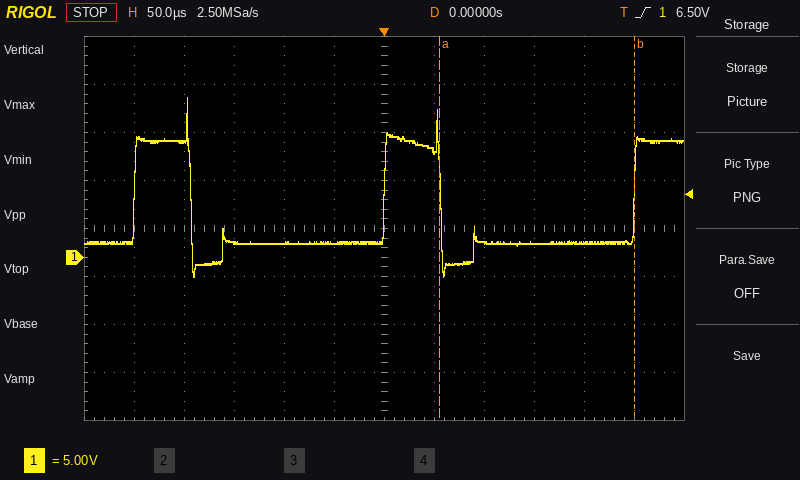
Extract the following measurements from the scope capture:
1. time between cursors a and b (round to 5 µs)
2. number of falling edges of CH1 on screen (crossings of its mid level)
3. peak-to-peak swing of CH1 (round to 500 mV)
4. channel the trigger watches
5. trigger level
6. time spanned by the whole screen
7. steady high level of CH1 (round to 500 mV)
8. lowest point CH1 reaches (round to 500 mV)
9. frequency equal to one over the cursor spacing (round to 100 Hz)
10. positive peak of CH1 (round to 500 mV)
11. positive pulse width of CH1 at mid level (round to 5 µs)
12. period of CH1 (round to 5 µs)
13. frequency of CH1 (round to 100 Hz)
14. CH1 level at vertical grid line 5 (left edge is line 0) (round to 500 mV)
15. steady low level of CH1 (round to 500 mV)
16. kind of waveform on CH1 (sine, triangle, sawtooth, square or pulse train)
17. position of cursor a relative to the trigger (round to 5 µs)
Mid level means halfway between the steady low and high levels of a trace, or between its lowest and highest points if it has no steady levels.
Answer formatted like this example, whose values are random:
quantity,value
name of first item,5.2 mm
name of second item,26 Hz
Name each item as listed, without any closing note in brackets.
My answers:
quantity,value
time between cursors a and b,195 µs
number of falling edges of CH1 on screen,2
peak-to-peak swing of CH1,18.5 V
channel the trigger watches,CH1
trigger level,6.50 V
time spanned by the whole screen,600 µs
steady high level of CH1,12.0 V
lowest point CH1 reaches,-2.0 V
frequency equal to one over the cursor spacing,5.1 kHz
positive peak of CH1,16.5 V
positive pulse width of CH1 at mid level,55 µs
period of CH1,250 µs
frequency of CH1,4.0 kHz
CH1 level at vertical grid line 5 (left edge is line 0),1.5 V
steady low level of CH1,1.5 V
kind of waveform on CH1,pulse train
position of cursor a relative to the trigger,+55 µs
